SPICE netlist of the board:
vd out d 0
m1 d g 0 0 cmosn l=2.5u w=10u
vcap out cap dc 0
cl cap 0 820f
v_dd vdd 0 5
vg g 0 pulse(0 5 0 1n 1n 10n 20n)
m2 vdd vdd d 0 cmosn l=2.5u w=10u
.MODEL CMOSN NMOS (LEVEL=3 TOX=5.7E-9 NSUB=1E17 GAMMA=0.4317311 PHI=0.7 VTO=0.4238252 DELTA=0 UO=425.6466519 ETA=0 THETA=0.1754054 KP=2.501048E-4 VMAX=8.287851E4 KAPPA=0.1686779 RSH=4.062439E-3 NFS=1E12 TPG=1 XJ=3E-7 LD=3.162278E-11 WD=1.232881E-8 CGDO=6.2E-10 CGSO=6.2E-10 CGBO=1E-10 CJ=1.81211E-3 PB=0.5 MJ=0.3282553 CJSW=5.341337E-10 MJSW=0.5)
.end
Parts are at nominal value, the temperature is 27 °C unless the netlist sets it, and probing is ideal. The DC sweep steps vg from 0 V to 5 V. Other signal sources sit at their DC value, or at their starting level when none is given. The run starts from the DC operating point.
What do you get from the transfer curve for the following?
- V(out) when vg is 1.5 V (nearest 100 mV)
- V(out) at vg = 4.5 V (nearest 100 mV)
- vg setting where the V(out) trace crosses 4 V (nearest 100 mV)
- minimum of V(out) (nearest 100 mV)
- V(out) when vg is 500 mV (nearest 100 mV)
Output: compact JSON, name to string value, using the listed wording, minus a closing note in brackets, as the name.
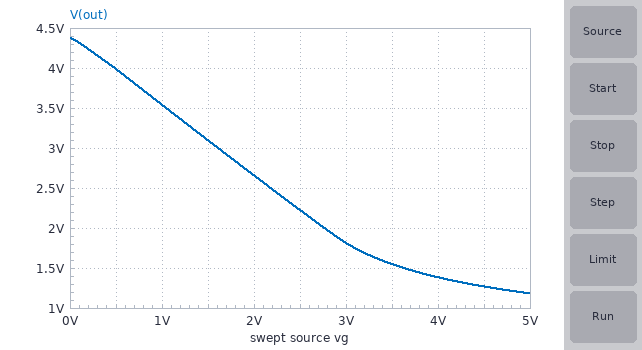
{"V(out) when vg is 1.5 V": "3.1 V", "V(out) at vg = 4.5 V": "1.3 V", "vg setting where the V(out) trace crosses 4 V": "500 mV", "minimum of V(out)": "1.2 V", "V(out) when vg is 500 mV": "4.0 V"}
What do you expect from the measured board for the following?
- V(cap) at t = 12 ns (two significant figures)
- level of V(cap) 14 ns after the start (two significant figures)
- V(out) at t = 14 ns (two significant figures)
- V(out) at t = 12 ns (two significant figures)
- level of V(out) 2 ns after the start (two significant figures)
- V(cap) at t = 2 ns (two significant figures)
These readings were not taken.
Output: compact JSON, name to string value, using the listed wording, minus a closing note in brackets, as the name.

{"V(cap) at t = 12 ns": "2.0 V", "level of V(cap) 14 ns after the start": "3.3 V", "V(out) at t = 14 ns": "3.3 V", "V(out) at t = 12 ns": "2.0 V", "level of V(out) 2 ns after the start": "1.4 V", "V(cap) at t = 2 ns": "1.4 V"}
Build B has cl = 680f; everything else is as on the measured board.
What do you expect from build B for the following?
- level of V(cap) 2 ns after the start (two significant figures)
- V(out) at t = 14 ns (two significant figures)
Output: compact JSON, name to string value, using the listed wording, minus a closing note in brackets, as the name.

{"level of V(cap) 2 ns after the start": "1.3 V", "V(out) at t = 14 ns": "3.4 V"}
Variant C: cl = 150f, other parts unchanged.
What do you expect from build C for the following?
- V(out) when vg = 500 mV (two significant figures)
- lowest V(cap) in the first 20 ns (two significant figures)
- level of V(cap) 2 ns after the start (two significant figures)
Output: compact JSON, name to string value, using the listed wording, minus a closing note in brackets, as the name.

{"V(out) when vg = 500 mV": "4.0 V", "lowest V(cap) in the first 20 ns": "1.1 V", "level of V(cap) 2 ns after the start": "1.2 V"}
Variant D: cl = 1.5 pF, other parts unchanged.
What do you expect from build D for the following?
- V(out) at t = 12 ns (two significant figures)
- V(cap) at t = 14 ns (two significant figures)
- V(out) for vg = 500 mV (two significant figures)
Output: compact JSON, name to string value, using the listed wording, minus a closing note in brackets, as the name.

{"V(out) at t = 12 ns": "1.7 V", "V(cap) at t = 14 ns": "2.9 V", "V(out) for vg = 500 mV": "4.0 V"}
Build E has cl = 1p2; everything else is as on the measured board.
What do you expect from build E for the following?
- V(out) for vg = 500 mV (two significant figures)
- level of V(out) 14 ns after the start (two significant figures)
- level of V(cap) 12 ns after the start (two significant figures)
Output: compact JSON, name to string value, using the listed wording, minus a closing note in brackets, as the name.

{"V(out) for vg = 500 mV": "4.0 V", "level of V(out) 14 ns after the start": "3.1 V", "level of V(cap) 12 ns after the start": "1.8 V"}
